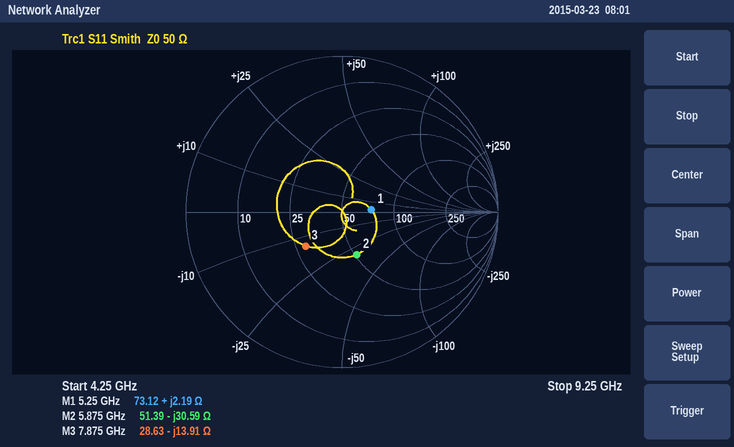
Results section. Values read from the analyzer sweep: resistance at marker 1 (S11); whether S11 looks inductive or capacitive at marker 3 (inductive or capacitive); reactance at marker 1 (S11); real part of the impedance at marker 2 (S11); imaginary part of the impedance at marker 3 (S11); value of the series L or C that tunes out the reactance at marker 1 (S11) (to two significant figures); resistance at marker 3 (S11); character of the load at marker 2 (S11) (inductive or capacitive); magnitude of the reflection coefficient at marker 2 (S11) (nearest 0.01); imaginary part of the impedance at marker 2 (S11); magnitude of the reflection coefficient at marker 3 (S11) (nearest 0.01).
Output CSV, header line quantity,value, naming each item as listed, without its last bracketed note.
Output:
quantity,value
resistance at marker 1,73.12 Ω
whether S11 looks inductive or capacitive at marker 3,capacitive
reactance at marker 1,+2.19 Ω
real part of the impedance at marker 2,51.39 Ω
imaginary part of the impedance at marker 3,-13.91 Ω
value of the series L or C that tunes out the reactance at marker 1 (S11),14 pF
resistance at marker 3,28.63 Ω
character of the load at marker 2 (S11),capacitive
magnitude of the reflection coefficient at marker 2 (S11),0.29
imaginary part of the impedance at marker 2,-30.59 Ω
magnitude of the reflection coefficient at marker 3 (S11),0.32
